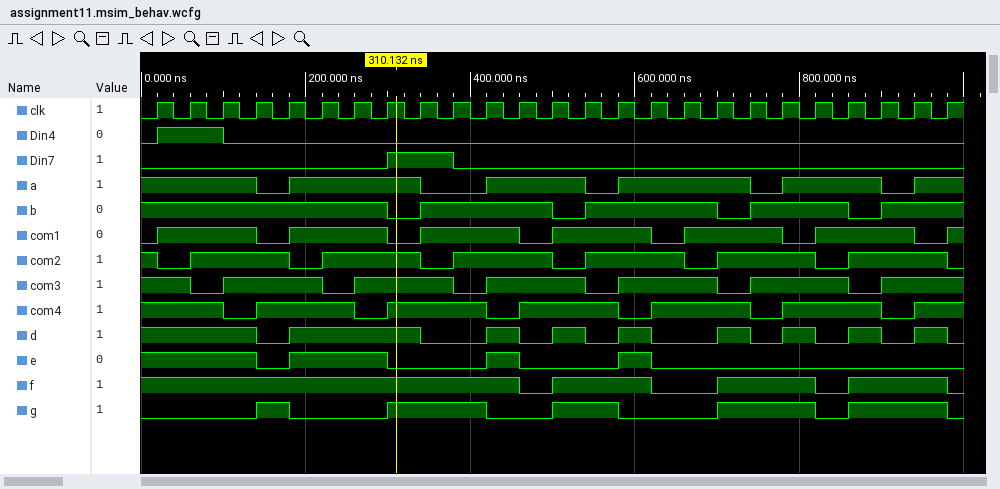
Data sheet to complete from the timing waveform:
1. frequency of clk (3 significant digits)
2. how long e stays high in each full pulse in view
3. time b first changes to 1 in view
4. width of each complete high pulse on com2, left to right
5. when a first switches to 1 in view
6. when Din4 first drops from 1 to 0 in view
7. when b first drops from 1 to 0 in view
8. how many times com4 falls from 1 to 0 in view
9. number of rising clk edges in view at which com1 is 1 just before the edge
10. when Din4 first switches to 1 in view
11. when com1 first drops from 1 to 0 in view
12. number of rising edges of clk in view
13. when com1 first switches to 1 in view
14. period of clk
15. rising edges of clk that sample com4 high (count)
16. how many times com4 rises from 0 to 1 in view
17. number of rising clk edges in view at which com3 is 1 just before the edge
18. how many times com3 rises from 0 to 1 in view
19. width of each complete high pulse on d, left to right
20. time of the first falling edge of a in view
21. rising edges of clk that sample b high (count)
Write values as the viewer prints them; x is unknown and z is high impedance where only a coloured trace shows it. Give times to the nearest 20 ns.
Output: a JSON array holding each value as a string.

["25.0 MHz", "120 ns, 40 ns, 40 ns", "340 ns", "120 ns, 120 ns, 120 ns, 120 ns, 120 ns, 120 ns", "180 ns", "100 ns", "300 ns", "6", "18", "20 ns", "140 ns", "25", "20 ns", "40 ns", "19", "6", "19", "6", "160 ns, 40 ns, 40 ns, 40 ns, 40 ns, 40 ns, 40 ns, 40 ns", "140 ns", "21"]
